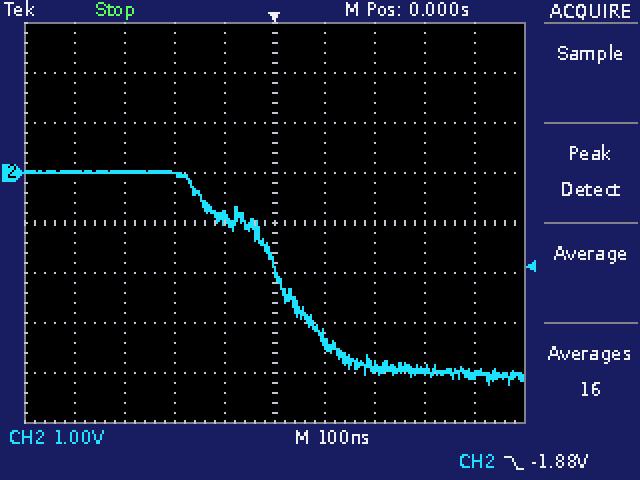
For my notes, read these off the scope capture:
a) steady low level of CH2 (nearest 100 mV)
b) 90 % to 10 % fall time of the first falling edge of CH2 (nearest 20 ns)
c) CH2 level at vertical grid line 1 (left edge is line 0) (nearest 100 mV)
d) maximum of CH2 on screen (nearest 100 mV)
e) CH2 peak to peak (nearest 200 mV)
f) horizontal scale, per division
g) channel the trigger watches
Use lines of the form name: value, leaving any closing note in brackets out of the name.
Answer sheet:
steady low level of CH2: -4.0 V
90 % to 10 % fall time of the first falling edge of CH2: 280 ns
CH2 level at vertical grid line 1 (left edge is line 0): 0.0 V
maximum of CH2 on screen: 0.0 V
CH2 peak to peak: 4.2 V
horizontal scale, per division: 100 ns
channel the trigger watches: CH2
